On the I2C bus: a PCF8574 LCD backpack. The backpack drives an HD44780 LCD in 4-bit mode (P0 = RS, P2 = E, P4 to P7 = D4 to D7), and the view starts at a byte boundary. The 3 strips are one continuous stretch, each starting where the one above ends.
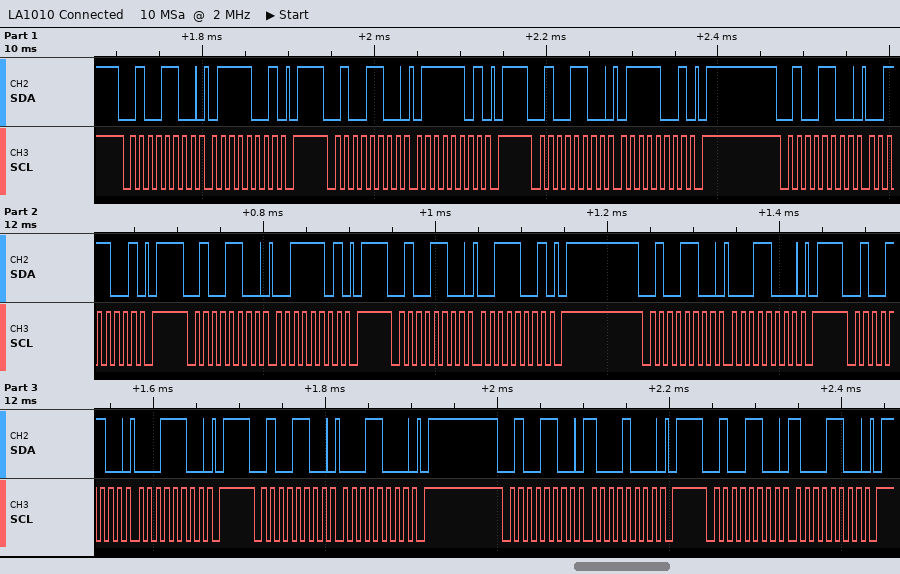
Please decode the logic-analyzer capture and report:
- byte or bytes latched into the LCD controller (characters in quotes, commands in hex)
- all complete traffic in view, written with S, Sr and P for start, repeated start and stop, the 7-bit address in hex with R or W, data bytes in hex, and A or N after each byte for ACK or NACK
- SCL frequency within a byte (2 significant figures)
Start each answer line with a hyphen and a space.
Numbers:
- 's'
- S 26W A 79 A P S 26W A 7D A P S 26W A 79 A P S 26W A 39 A P S 26W A 3D A P S 26W A 39 A P S 26W A 18 A P S 26W A 1C A P S 26W A 18 A P S 26W A 88 A P S 26W A 8C A P
- 100 kHz
